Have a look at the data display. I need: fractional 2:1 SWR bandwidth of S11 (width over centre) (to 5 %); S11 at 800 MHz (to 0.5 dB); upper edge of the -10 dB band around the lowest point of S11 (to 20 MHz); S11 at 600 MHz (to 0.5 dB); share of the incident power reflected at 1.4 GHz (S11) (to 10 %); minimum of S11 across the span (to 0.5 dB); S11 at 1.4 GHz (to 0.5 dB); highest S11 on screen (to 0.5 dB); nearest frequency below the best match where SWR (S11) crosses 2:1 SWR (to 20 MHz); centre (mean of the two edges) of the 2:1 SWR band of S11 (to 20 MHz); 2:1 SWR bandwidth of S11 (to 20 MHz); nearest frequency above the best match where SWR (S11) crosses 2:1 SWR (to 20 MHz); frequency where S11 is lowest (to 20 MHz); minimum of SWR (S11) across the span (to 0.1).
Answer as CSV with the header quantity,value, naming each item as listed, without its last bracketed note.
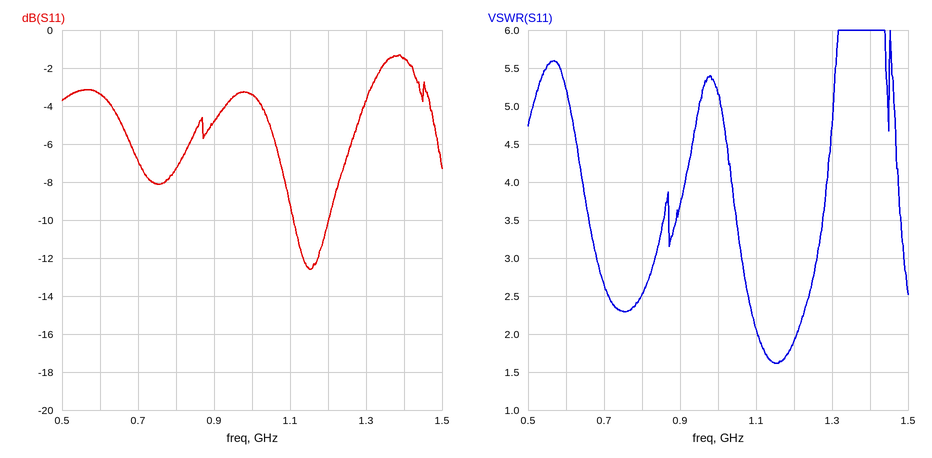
quantity,value
fractional 2:1 SWR bandwidth of S11 (width over centre),10 %
S11 at 800 MHz,-7.5 dB
upper edge of the -10 dB band around the lowest point of S11,1.20 GHz
S11 at 600 MHz,-3.5 dB
share of the incident power reflected at 1.4 GHz (S11),70 %
minimum of S11 across the span,-12.5 dB
S11 at 1.4 GHz,-1.5 dB
highest S11 on screen,-1.5 dB
nearest frequency below the best match where SWR (S11) crosses 2:1 SWR,1.10 GHz
centre (mean of the two edges) of the 2:1 SWR band of S11,1.16 GHz
2:1 SWR bandwidth of S11,100 MHz
nearest frequency above the best match where SWR (S11) crosses 2:1 SWR,1.20 GHz
frequency where S11 is lowest,1.16 GHz
minimum of SWR (S11) across the span,1.6
